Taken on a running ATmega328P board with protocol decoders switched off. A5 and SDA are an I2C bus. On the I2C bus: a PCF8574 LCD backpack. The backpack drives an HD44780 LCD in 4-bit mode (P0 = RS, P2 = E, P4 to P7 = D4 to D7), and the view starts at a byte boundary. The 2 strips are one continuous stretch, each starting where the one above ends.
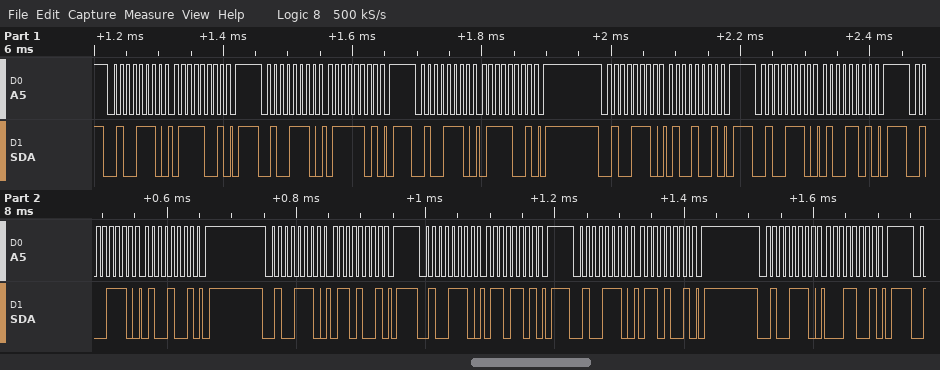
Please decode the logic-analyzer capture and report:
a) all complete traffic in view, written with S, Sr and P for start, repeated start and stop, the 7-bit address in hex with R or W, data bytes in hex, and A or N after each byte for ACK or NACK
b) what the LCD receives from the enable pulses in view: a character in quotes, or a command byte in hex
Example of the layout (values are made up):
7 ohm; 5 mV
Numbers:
S 27W A 79 A P S 27W A 7D A P S 27W A 79 A P S 27W A 49 A P S 27W A 4D A P S 27W A 49 A P S 27W A 69 A P S 27W A 6D A P S 27W A 69 A P S 27W A 19 A P; 't'
